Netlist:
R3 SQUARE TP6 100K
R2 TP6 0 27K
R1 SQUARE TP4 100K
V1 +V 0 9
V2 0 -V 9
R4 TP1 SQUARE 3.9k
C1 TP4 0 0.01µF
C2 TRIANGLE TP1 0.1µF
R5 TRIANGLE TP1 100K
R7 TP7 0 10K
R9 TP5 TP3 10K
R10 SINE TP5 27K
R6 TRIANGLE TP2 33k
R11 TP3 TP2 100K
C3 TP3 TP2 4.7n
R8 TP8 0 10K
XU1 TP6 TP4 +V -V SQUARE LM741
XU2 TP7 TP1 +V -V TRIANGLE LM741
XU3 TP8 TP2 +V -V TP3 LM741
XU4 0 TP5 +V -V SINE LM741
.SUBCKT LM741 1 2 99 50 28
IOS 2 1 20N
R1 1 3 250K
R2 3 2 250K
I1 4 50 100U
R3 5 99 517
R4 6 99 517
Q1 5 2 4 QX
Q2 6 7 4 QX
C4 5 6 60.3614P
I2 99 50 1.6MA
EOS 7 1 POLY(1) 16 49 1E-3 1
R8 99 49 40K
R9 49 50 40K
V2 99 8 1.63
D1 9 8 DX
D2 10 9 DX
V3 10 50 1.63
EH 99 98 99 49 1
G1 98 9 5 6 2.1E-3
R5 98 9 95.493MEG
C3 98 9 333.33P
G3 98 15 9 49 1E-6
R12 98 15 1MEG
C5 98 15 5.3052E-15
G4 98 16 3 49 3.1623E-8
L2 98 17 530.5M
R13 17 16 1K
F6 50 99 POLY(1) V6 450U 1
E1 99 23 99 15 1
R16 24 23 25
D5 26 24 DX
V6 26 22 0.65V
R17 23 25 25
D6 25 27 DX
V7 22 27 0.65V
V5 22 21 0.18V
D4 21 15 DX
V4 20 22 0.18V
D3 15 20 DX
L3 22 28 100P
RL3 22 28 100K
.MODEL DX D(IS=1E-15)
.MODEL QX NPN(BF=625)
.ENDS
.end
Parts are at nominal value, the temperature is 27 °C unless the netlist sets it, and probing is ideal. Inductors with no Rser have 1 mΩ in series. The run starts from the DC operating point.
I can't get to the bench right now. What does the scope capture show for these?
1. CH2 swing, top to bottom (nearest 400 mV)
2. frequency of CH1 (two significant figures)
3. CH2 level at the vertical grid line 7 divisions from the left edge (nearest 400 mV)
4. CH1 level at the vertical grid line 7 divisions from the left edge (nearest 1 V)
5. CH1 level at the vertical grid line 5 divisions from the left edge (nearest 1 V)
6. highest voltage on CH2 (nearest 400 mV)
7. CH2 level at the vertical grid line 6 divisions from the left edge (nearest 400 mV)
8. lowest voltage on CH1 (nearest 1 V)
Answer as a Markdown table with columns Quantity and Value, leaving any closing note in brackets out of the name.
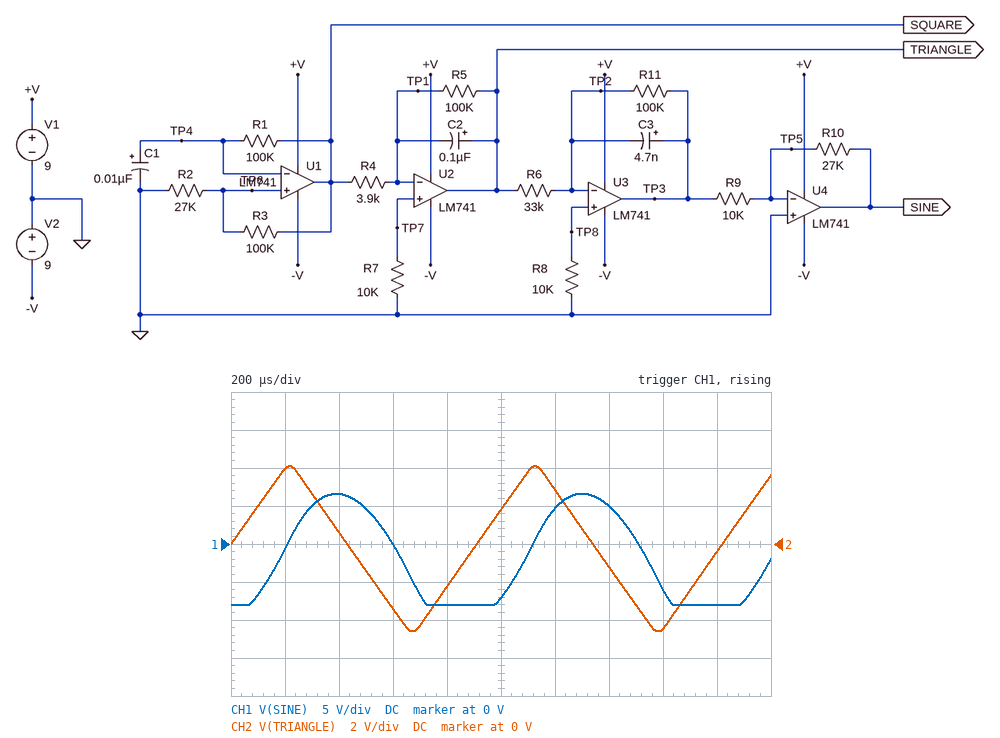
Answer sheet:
| Quantity | Value |
|---|---|
| CH2 swing, top to bottom | 8.8 V |
| frequency of CH1 | 1.1 kHz |
| CH2 level at the vertical grid line 7 divisions from the left edge | -1.2 V |
| CH1 level at the vertical grid line 7 divisions from the left edge | 5 V |
| CH1 level at the vertical grid line 5 divisions from the left edge | -7 V |
| highest voltage on CH2 | 4.0 V |
| CH2 level at the vertical grid line 6 divisions from the left edge | 2.8 V |
| lowest voltage on CH1 | -8 V |
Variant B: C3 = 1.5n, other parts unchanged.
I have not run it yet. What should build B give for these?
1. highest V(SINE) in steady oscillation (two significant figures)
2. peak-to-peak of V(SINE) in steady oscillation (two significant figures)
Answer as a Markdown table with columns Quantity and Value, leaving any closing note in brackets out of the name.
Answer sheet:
| Quantity | Value |
|---|---|
| highest V(SINE) in steady oscillation | 8.0 V |
| peak-to-peak of V(SINE) in steady oscillation | 16 V |
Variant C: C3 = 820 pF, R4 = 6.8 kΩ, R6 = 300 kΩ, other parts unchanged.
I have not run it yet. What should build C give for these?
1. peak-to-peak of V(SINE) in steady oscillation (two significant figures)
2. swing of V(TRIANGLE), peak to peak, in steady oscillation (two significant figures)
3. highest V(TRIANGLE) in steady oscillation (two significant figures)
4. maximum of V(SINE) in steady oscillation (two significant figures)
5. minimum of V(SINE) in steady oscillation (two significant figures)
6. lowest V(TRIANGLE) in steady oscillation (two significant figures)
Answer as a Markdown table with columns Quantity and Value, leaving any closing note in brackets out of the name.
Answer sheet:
| Quantity | Value |
|---|---|
| peak-to-peak of V(SINE) in steady oscillation | 3.6 V |
| swing of V(TRIANGLE), peak to peak, in steady oscillation | 5.0 V |
| highest V(TRIANGLE) in steady oscillation | 2.4 V |
| maximum of V(SINE) in steady oscillation | 1.7 V |
| minimum of V(SINE) in steady oscillation | -1.9 V |
| lowest V(TRIANGLE) in steady oscillation | -2.6 V |
